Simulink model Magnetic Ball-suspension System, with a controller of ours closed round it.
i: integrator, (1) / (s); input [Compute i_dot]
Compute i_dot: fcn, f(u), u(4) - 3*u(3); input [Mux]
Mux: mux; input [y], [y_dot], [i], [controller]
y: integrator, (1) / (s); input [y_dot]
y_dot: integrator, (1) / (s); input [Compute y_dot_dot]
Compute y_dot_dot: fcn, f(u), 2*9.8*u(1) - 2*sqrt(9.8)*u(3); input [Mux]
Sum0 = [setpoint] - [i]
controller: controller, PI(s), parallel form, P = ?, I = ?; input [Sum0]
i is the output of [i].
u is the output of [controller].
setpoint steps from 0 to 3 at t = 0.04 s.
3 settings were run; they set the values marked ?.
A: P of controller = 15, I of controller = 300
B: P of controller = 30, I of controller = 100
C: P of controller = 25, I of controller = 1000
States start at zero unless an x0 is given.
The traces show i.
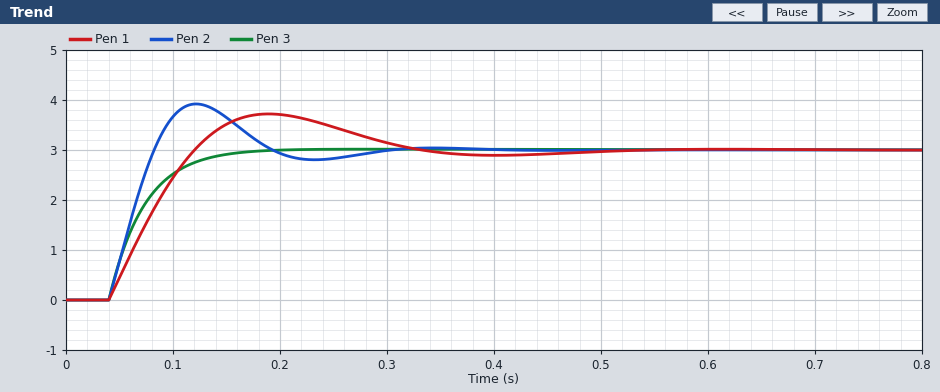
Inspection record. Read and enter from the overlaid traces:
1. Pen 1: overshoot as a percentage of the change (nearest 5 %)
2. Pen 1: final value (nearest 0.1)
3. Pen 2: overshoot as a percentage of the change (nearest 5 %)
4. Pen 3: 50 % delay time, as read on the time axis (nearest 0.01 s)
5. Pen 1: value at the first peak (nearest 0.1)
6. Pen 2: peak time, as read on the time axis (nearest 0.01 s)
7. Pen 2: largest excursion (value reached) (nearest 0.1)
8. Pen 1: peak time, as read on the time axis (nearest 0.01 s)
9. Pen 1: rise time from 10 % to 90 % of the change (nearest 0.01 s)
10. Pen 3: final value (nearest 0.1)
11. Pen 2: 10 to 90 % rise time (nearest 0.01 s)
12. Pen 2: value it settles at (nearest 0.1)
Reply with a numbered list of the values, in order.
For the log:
1. 25 %
2. 3.0
3. 30 %
4. 0.06 s
5. 3.7
6. 0.12 s
7. 3.9
8. 0.19 s
9. 0.06 s
10. 3.0
11. 0.03 s
12. 3.0
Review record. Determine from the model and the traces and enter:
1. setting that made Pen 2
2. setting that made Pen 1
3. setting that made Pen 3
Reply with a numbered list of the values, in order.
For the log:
1. C
2. A
3. B
